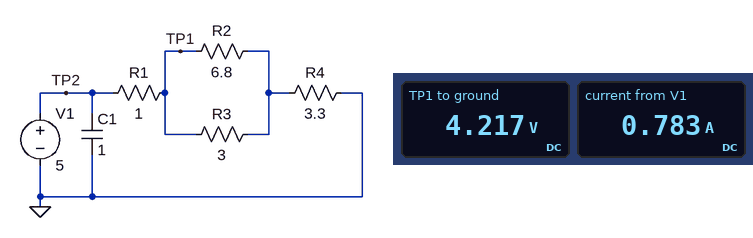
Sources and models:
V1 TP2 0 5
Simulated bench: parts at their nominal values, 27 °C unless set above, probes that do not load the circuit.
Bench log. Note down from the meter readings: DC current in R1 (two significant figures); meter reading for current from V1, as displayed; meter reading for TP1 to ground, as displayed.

780 mA
0.783 A
4.217 V
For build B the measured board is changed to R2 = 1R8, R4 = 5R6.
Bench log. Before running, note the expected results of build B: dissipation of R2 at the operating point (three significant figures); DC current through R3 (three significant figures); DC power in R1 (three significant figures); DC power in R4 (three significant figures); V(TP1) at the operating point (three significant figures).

295 mW
243 mA
419 mW
2.35 W
4.35 V
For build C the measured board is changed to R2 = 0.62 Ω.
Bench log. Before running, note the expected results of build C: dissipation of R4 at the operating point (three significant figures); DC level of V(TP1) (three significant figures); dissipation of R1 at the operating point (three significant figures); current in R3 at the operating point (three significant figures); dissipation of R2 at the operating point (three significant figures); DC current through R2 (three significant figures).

3.56 W
3.96 V
1.08 W
178 mA
459 mW
861 mA
